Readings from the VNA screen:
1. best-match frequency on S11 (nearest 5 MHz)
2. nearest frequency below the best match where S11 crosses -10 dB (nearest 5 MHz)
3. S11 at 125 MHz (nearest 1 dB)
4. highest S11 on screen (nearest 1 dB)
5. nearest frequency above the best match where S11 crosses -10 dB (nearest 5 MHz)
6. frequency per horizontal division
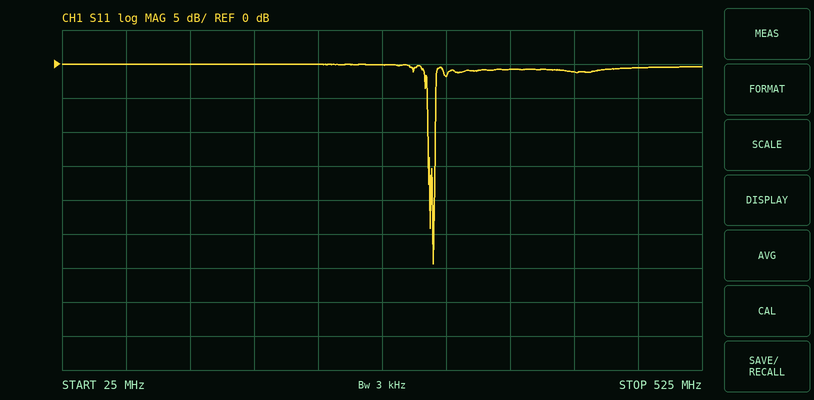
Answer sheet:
315 MHz
310 MHz
0 dB
0 dB
315 MHz
50 MHz
